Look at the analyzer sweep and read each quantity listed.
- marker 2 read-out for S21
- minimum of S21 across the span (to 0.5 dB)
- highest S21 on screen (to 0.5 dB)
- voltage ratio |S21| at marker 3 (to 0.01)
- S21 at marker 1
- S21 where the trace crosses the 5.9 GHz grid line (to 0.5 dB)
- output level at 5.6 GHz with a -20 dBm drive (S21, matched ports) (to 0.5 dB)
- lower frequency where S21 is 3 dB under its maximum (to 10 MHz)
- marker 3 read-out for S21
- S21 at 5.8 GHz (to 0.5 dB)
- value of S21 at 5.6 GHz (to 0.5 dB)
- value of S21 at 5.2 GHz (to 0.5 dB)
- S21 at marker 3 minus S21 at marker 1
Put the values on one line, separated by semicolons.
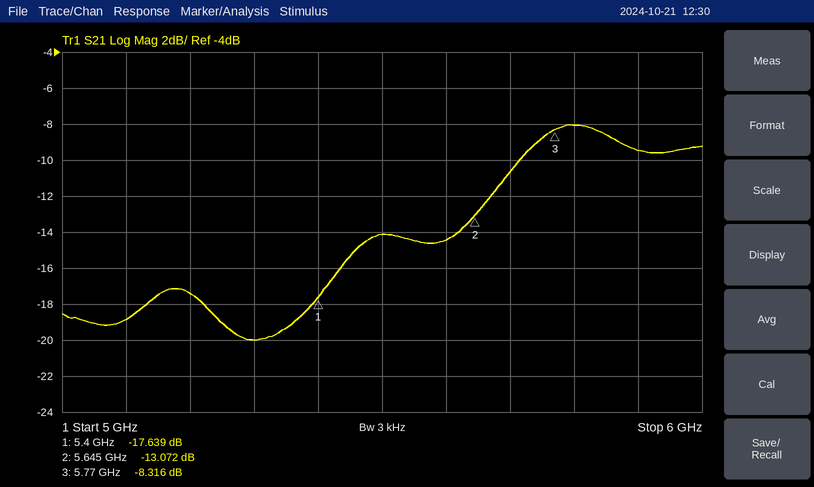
-13.072 dB; -20.0 dB; -8.0 dB; 0.38; -17.639 dB; -9.5 dB; -34.5 dBm; 5.69 GHz; -8.316 dB; -8.0 dB; -14.5 dB; -17.5 dB; 9.323 dB
